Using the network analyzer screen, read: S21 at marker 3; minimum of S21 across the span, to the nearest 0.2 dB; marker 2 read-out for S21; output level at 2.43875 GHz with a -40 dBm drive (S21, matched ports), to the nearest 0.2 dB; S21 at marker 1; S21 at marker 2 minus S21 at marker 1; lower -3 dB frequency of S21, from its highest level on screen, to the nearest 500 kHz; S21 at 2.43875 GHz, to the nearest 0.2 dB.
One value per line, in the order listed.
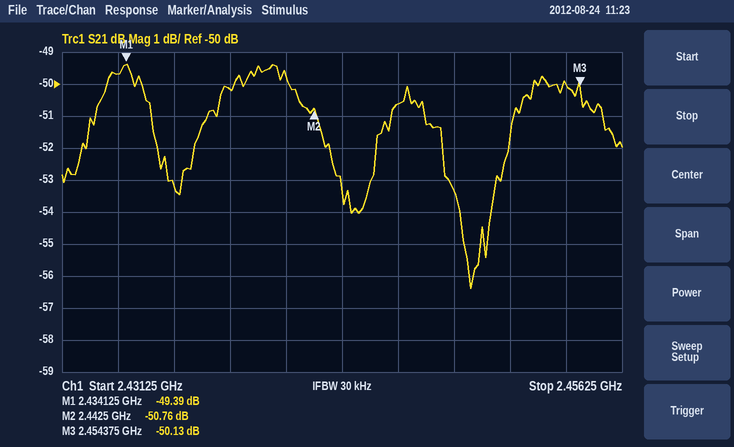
-50.13 dB
-56.4 dB
-50.76 dB
-90.2 dBm
-49.39 dB
-1.37 dB
2.4320 GHz
-50.2 dB
